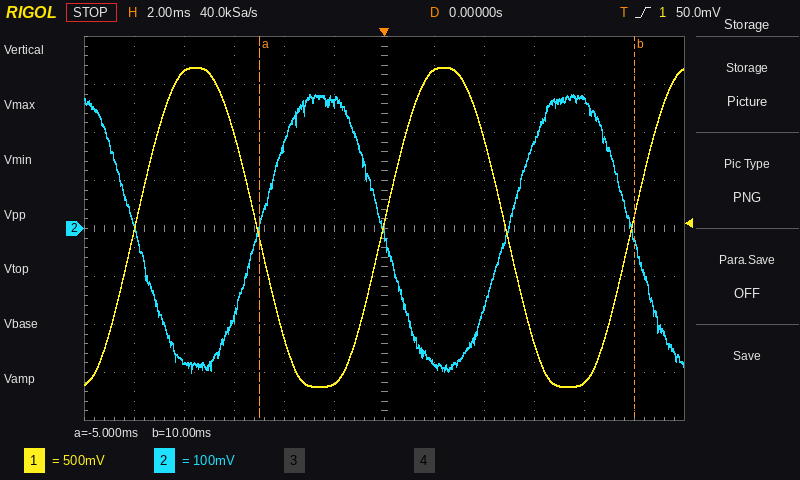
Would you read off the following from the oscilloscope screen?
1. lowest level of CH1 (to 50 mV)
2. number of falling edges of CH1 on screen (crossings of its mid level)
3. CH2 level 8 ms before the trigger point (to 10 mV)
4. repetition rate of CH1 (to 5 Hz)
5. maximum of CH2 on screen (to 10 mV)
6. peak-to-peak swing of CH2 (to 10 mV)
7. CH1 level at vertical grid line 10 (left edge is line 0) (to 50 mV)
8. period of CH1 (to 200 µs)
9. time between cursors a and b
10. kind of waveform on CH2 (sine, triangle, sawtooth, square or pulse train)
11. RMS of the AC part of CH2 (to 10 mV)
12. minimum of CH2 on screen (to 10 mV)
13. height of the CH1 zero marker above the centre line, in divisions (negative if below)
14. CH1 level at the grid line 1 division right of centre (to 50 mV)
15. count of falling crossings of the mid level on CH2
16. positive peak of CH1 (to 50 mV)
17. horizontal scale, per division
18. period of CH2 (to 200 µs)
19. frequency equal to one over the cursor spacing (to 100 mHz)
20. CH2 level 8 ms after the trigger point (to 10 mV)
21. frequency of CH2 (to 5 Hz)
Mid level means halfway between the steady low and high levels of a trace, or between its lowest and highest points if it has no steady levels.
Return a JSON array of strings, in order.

["-1.65 V", "2", "-280 mV", "100 Hz", "280 mV", "580 mV", "-1.60 V", "10.0 ms", "15.0 ms", "sine", "210 mV", "-300 mV", "0.0 div", "1.65 V", "3", "1.70 V", "2 ms", "10.0 ms", "66.7 Hz", "270 mV", "100 Hz"]
